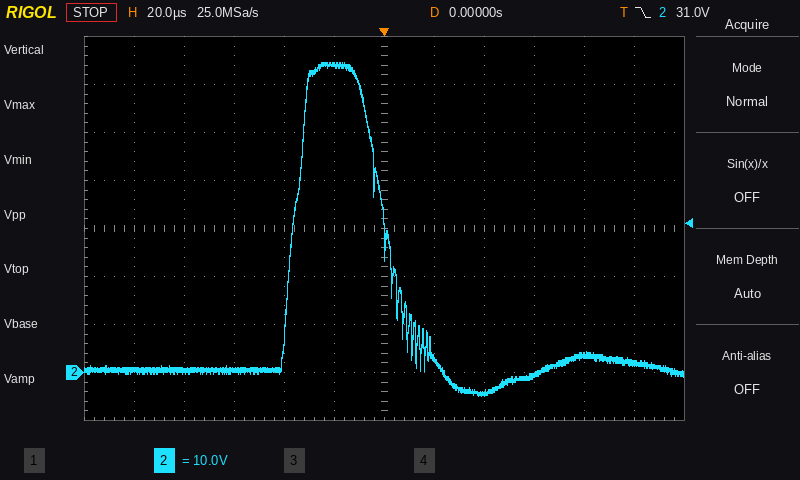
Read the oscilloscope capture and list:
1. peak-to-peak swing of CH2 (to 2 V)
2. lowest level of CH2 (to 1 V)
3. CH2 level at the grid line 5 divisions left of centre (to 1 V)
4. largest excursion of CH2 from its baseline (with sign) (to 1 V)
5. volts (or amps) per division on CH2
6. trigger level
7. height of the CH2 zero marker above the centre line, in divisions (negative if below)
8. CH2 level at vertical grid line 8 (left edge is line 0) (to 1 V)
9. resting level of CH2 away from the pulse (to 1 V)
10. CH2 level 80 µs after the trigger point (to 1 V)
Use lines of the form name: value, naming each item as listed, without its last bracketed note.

peak-to-peak swing of CH2: 70 V
lowest level of CH2: -5 V
CH2 level at the grid line 5 divisions left of centre: 1 V
largest excursion of CH2 from its baseline (with sign): +64 V
volts (or amps) per division on CH2: 10 V
trigger level: 31.0 V
height of the CH2 zero marker above the centre line, in divisions: -3.0 div
CH2 level at vertical grid line 8 (left edge is line 0): -4 V
resting level of CH2 away from the pulse: 1 V
CH2 level 80 µs after the trigger point: 4 V
